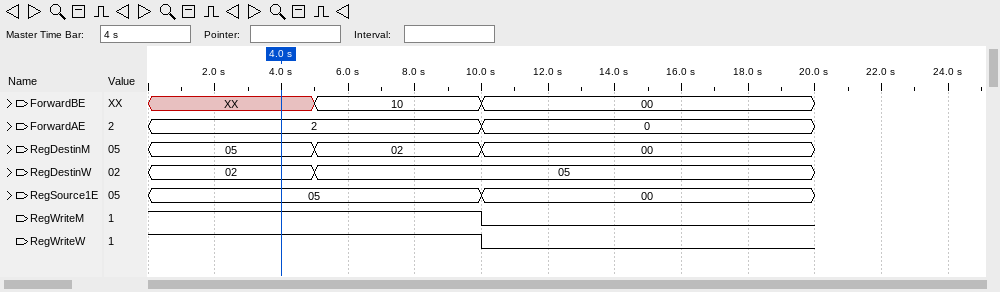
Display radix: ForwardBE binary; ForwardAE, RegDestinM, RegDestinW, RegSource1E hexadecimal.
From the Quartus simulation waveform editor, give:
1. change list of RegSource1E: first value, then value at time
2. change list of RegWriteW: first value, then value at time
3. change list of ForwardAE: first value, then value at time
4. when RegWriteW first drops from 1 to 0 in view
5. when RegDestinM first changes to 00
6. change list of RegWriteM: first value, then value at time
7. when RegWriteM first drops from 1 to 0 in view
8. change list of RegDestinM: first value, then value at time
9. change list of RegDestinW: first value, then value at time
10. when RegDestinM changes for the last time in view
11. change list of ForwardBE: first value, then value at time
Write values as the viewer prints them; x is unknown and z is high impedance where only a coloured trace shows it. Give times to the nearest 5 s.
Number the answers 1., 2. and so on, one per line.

1. 05, 00 at 10 s
2. 1, 0 at 10 s
3. 2, 0 at 10 s
4. 10 s
5. 10 s
6. 1, 0 at 10 s
7. 10 s
8. 05, 02 at 5 s, 00 at 10 s
9. 02, 05 at 5 s
10. 10 s
11. XX, 10 at 5 s, 00 at 10 s
